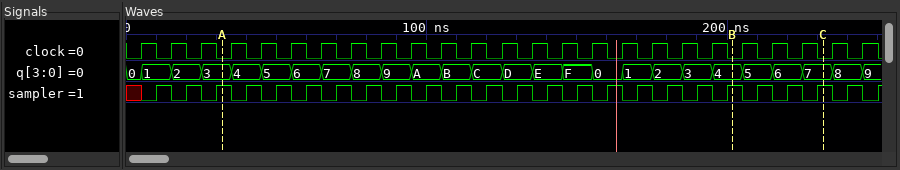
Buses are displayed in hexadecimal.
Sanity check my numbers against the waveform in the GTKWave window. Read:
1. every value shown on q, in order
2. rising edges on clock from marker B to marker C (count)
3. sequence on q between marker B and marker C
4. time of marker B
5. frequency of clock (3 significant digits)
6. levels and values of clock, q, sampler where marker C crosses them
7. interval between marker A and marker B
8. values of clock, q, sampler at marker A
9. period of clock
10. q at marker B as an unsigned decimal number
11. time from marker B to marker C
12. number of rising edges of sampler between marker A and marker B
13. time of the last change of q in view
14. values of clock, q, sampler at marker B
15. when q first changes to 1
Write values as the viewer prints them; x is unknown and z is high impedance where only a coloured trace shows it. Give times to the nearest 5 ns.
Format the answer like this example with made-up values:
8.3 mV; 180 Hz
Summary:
0, 1, 2, 3, 4, 5, 6, 7, 8, 9, A, B, C, D, E, F, 0, 1, 2, 3, 4, 5, 6, 7, 8, 9; 3; 4, 5, 6, 7; 200 ns; 100 MHz; clock=0, q=7, sampler=1; 170 ns; clock=0, q=3, sampler=1; 10 ns; 4; 30 ns; 17; 245 ns; clock=0, q=4, sampler=1; 5 ns
